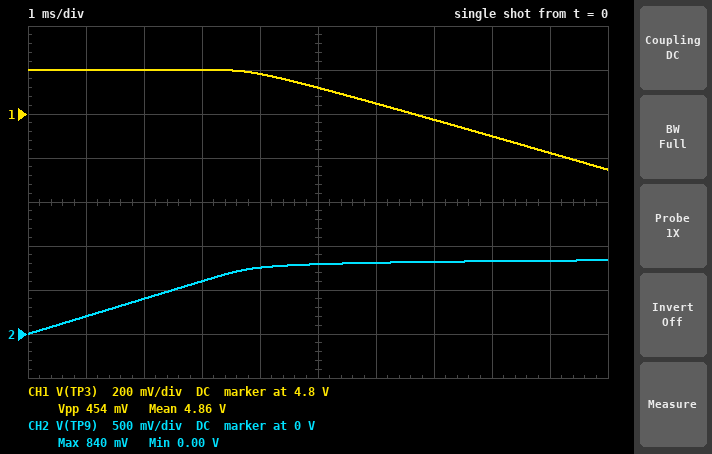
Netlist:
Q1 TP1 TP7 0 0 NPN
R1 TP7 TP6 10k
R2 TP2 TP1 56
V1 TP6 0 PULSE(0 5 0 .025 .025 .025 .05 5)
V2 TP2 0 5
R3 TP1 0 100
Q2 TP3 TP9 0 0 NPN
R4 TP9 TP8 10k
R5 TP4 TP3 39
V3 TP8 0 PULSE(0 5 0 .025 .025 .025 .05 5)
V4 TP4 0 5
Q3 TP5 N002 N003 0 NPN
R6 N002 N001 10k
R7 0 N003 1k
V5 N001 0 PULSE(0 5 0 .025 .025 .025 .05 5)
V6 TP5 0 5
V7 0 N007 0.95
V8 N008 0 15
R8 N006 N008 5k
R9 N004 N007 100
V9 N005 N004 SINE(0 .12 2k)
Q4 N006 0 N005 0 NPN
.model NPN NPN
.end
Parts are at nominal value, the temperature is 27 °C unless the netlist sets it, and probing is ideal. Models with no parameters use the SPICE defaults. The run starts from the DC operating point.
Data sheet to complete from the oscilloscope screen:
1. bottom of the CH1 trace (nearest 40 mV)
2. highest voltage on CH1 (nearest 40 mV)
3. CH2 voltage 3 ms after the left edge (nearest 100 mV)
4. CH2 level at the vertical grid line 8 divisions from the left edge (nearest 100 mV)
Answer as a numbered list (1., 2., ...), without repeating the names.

1. 4.56 V
2. 5.00 V
3. 600 mV
4. 800 mV
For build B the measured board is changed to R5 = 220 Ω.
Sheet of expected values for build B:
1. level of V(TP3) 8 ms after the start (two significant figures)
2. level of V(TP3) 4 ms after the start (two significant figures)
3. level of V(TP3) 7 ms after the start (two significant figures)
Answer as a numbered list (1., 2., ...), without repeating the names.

1. 3.3 V
2. 4.9 V
3. 3.7 V
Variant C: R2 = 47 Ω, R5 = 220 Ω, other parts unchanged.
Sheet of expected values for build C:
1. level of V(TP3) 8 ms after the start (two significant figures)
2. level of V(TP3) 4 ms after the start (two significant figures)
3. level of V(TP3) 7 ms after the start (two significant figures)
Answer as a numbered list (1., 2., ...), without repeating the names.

1. 3.3 V
2. 4.9 V
3. 3.7 V
